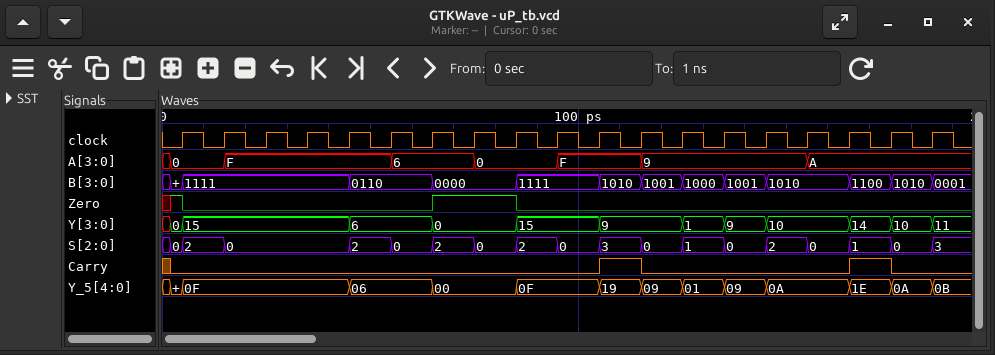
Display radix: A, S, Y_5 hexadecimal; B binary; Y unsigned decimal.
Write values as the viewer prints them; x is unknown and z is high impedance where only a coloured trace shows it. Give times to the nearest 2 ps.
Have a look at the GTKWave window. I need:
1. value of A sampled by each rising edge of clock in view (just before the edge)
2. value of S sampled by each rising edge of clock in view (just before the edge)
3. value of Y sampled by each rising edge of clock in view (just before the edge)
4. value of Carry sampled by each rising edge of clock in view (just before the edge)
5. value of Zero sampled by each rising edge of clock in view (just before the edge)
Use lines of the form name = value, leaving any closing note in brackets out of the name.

value of A sampled by each rising edge of clock in view = 0, 0, F, F, F, F, 6, 6, 0, 0, F, F, 9, 9, 9, 9, A, A, A
value of S sampled by each rising edge of clock in view = 0, 2, 0, 0, 0, 2, 0, 2, 0, 2, 0, 3, 0, 1, 0, 2, 0, 1, 0
value of Y sampled by each rising edge of clock in view = 0, 15, 15, 15, 15, 6, 6, 0, 0, 15, 15, 9, 9, 1, 9, 10, 10, 14, 10
value of Carry sampled by each rising edge of clock in view = 0 0 0 0 0 0 0 0 0 0 0 1 0 0 0 0 0 1 0
value of Zero sampled by each rising edge of clock in view = 1 0 0 0 0 0 0 1 1 0 0 0 0 0 0 0 0 0 0
